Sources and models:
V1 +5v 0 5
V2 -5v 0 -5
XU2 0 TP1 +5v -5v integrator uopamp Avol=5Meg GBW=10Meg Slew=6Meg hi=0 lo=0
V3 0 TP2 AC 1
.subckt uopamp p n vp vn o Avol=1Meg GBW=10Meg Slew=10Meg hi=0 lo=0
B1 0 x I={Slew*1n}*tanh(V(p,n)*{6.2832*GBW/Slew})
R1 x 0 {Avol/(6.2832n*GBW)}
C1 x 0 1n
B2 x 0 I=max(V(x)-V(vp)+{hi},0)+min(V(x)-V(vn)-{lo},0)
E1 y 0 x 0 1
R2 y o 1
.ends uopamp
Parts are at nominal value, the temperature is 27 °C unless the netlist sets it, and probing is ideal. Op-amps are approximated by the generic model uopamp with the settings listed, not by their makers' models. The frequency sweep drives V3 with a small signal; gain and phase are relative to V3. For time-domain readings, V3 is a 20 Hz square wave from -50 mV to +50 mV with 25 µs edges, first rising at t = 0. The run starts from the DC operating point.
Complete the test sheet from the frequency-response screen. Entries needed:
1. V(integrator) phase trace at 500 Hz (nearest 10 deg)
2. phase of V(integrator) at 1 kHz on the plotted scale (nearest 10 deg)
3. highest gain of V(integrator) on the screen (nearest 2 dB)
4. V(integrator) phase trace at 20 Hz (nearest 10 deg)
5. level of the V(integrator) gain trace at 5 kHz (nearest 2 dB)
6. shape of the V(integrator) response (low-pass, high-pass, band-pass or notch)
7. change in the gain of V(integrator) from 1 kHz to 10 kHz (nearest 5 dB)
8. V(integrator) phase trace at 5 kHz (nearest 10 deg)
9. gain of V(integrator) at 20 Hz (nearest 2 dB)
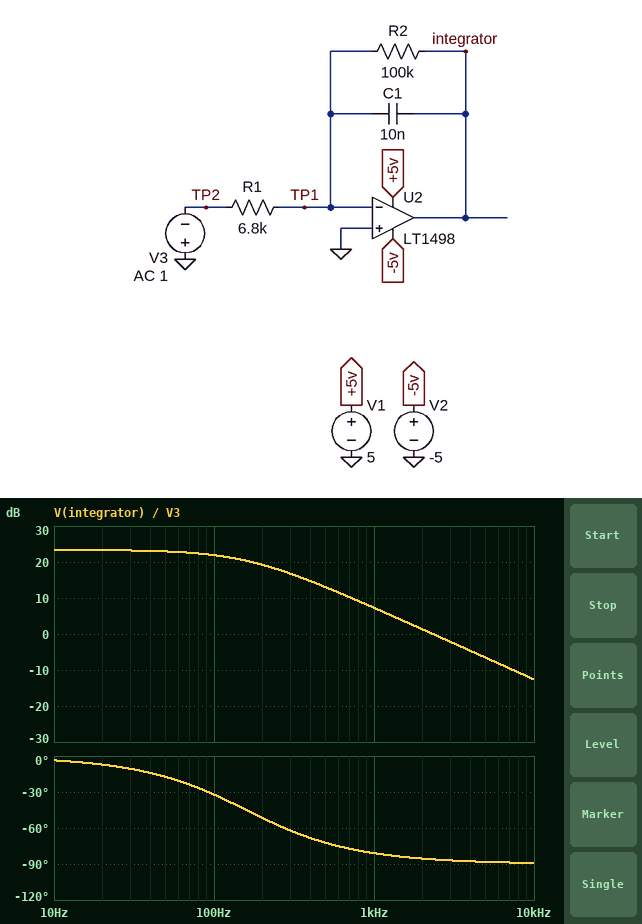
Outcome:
-70 deg
-80 deg
24 dB
-10 deg
-6 dB
low-pass
-20 dB
-90 deg
24 dB
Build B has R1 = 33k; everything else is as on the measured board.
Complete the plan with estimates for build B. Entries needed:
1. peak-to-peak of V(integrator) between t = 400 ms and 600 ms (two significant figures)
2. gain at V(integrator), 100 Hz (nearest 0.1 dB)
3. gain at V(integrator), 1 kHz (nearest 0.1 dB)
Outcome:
300 mV
8.2 dB
-6.4 dB
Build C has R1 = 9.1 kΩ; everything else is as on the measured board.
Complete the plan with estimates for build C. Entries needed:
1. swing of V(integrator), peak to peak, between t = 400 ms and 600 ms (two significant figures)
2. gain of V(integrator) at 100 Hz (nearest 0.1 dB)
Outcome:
1.1 V
19.4 dB
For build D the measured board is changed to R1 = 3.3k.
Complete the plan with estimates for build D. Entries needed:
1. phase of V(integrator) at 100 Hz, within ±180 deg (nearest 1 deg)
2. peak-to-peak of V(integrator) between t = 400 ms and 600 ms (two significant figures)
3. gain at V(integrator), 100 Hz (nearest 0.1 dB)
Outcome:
-32 deg
3.0 V
28.2 dB
